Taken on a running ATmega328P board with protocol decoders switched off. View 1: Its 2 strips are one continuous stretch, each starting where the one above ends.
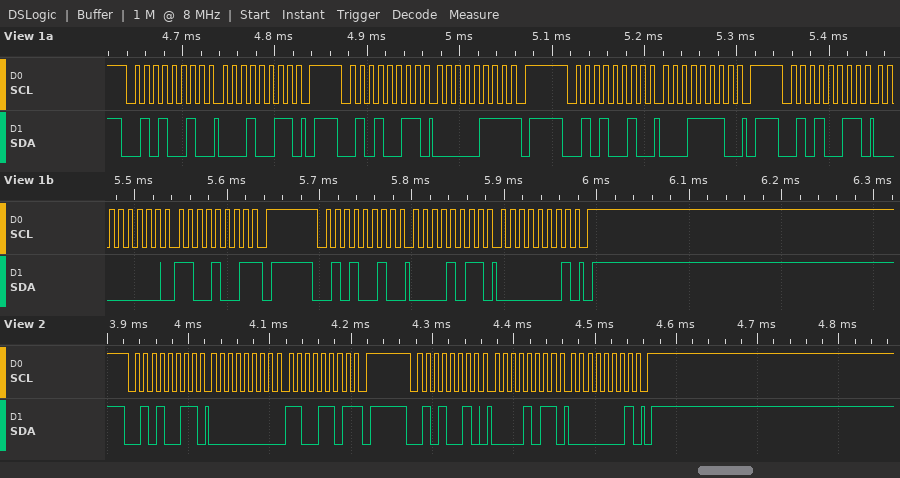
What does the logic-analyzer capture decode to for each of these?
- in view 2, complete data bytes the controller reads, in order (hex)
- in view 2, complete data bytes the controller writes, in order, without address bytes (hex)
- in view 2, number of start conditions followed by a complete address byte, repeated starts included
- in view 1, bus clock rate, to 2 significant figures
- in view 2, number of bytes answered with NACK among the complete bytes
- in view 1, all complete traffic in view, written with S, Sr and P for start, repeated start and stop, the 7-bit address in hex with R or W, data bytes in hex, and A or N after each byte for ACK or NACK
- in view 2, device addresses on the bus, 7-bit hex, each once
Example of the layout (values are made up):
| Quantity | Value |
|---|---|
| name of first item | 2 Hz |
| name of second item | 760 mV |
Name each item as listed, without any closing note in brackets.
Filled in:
| Quantity | Value |
|---|---|
| in view 2, complete data bytes the controller reads, in order | 00 CD |
| in view 2, complete data bytes the controller writes, in order, without address bytes | 0B 01 |
| in view 2, number of start conditions followed by a complete address byte, repeated starts included | 2 |
| in view 1, bus clock rate, to 2 significant figures | 100 kHz |
| in view 2, number of bytes answered with NACK among the complete bytes | 1 |
| in view 1, all complete traffic in view, written with S, Sr and P for start, repeated start and stop, the 7-bit address in hex with R or W, data bytes in hex, and A or N after each byte for ACK or NACK | S 29W A 13 A P S 29R A 07 N P S 29W A 1E A P S 29R A 00 A C9 N P S 29W A 0B A 01 A P |
| in view 2, device addresses on the bus, 7-bit hex, each once | 0x29 |
